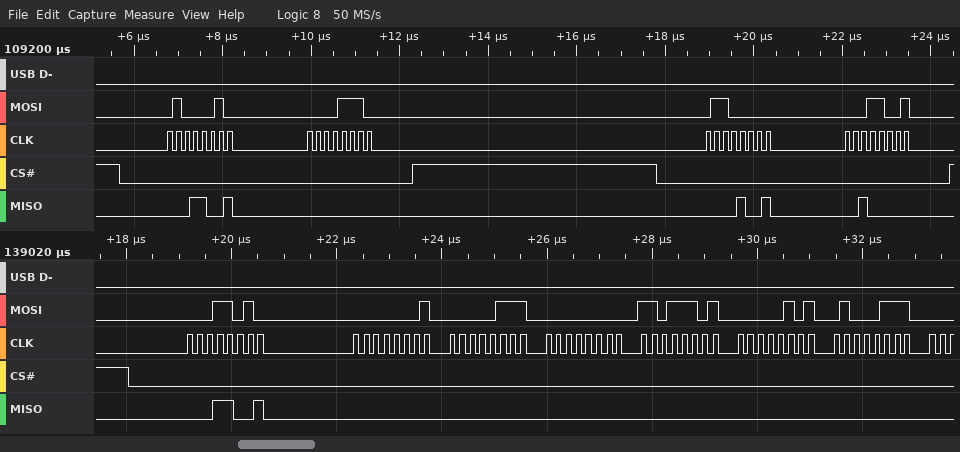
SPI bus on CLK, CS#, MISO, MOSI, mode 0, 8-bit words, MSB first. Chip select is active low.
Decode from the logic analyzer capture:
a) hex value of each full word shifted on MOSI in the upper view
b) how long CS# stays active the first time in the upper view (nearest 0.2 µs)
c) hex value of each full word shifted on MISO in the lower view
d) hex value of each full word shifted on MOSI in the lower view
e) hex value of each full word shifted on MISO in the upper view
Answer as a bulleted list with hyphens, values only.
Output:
- 42, 0E, 60, 19
- 6.6 µs
- 19, 00, 00, 00, 00, 00, 00
- 1A, 01, 07, 00, DD, 05, 47
- 19, 00, 09, 20
